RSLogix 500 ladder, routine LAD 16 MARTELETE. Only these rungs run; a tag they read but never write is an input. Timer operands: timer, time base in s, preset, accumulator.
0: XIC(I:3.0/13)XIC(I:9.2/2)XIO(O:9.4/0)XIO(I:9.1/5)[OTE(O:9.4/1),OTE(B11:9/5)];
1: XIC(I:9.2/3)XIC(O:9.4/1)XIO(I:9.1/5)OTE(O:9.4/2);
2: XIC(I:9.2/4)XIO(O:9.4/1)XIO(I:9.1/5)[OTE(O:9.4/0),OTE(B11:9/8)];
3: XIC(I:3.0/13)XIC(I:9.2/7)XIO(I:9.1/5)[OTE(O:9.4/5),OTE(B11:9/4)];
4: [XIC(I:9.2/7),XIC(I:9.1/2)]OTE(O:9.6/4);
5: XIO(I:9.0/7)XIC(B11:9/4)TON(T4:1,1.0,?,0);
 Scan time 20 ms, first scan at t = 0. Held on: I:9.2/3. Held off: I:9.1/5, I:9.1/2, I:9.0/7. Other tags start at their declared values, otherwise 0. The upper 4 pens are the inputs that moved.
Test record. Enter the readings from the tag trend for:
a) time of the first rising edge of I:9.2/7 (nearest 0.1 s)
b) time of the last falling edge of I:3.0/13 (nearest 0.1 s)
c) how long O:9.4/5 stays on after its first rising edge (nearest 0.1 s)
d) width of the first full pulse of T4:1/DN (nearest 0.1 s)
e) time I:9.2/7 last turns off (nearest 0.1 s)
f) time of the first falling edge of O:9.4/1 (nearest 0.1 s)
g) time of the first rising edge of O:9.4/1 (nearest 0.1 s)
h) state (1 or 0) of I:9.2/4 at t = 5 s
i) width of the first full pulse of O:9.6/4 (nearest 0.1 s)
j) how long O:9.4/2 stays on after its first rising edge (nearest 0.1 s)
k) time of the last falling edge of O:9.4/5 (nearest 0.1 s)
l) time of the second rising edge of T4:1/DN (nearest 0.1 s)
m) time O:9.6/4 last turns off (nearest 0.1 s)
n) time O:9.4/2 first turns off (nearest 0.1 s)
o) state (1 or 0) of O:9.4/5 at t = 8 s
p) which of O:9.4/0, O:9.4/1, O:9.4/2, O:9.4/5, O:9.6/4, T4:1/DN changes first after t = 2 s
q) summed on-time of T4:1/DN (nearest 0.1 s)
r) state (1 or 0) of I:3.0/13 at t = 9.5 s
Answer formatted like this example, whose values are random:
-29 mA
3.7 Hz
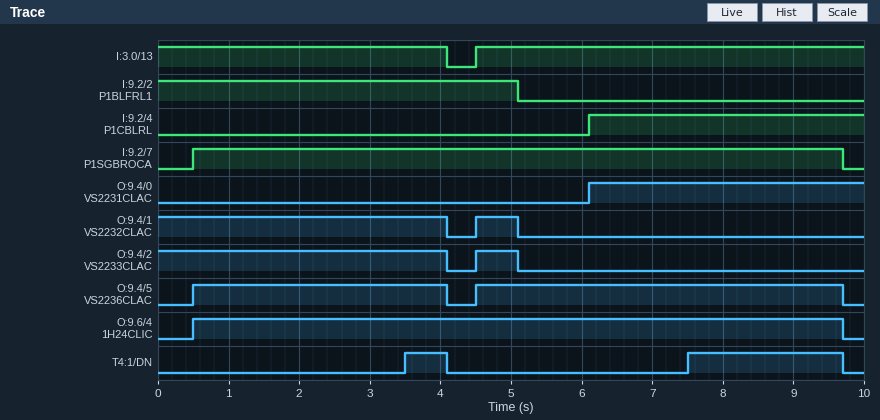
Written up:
0.5 s
4.1 s
3.6 s
0.6 s
9.7 s
4.1 s
4.5 s
0
9.2 s
0.6 s
9.7 s
7.5 s
9.7 s
4.1 s
1
T4:1/DN
2.8 s
1
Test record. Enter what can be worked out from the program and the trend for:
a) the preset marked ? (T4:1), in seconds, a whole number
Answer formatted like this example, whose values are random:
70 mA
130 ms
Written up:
3 s
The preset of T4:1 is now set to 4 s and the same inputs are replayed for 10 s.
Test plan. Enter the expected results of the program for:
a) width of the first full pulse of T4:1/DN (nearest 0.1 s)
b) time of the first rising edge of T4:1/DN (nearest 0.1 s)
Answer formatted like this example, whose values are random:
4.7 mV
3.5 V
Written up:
1.2 s
8.5 s
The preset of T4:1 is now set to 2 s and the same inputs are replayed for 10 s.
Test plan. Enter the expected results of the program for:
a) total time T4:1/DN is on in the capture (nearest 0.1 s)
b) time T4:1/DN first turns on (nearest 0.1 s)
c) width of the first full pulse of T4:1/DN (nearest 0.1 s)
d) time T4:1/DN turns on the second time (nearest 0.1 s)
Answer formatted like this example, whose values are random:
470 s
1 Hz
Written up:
4.8 s
2.5 s
1.6 s
6.5 s
